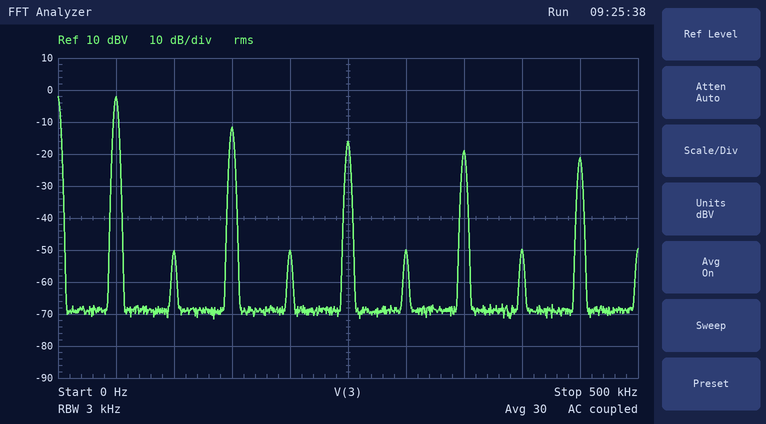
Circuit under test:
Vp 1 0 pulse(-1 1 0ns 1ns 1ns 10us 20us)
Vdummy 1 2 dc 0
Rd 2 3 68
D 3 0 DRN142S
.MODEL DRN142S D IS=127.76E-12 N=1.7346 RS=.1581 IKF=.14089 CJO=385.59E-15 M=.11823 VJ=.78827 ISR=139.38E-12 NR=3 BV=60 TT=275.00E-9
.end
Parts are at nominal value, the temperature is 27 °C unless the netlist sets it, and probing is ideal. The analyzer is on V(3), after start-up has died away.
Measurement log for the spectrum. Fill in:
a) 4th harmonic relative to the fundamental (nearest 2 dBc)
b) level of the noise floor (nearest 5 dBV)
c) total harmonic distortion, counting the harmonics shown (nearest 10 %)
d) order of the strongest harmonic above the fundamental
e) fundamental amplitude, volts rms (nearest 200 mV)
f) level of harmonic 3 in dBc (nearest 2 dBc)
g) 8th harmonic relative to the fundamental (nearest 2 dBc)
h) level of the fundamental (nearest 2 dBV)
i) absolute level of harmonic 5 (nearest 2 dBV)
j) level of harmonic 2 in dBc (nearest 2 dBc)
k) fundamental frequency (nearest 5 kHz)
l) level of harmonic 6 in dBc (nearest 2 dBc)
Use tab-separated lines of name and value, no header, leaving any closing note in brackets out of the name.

4th harmonic relative to the fundamental	-48 dBc
level of the noise floor	-70 dBV
total harmonic distortion, counting the harmonics shown	40 %
order of the strongest harmonic above the fundamental	3
fundamental amplitude, volts rms	800 mV
level of harmonic 3 in dBc	-10 dBc
8th harmonic relative to the fundamental	-48 dBc
level of the fundamental	-2 dBV
absolute level of harmonic 5	-16 dBV
level of harmonic 2 in dBc	-48 dBc
fundamental frequency	50 kHz
level of harmonic 6 in dBc	-48 dBc
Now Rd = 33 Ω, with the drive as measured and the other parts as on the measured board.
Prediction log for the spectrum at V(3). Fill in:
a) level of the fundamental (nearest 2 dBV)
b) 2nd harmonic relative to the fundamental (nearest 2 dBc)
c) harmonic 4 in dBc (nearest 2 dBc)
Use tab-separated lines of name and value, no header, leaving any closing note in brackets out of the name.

level of the fundamental	-2 dBV
2nd harmonic relative to the fundamental	-50 dBc
harmonic 4 in dBc	-50 dBc
